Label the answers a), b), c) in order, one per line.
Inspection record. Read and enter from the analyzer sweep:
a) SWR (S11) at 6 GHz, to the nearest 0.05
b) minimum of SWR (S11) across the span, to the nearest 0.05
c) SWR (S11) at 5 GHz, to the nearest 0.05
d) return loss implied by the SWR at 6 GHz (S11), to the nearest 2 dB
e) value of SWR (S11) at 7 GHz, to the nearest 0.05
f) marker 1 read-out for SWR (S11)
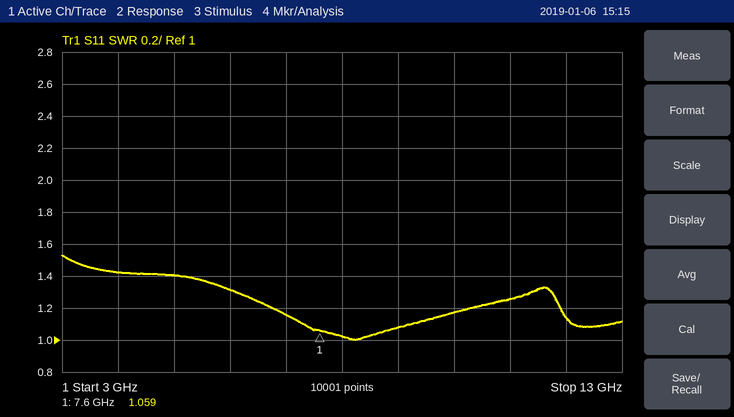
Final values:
a) 1.30
b) 1.00
c) 1.40
d) 18 dB
e) 1.15
f) 1.059
